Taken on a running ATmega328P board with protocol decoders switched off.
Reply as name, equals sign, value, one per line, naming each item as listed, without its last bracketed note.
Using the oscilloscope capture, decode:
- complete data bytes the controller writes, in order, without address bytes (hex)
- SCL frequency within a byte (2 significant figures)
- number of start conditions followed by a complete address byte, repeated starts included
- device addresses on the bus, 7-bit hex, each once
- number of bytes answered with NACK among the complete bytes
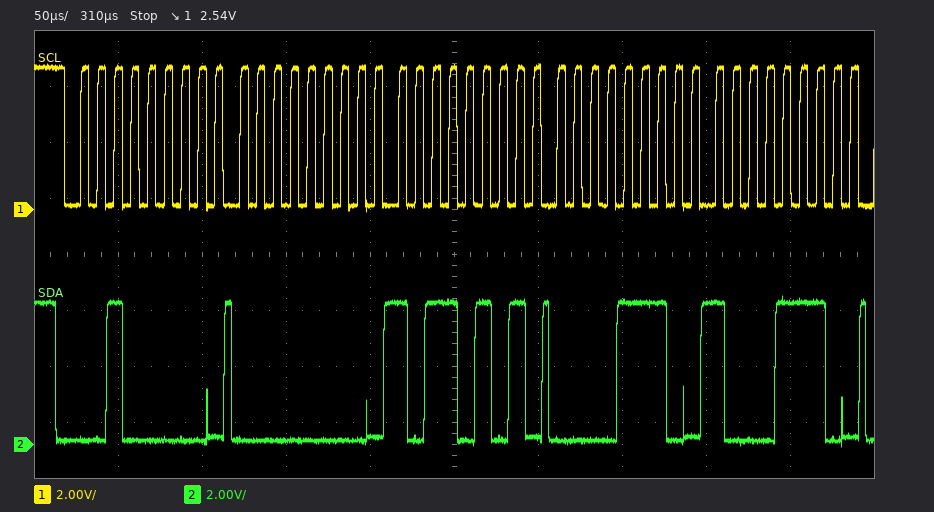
complete data bytes the controller writes, in order, without address bytes = 00 B5 0E 8E
SCL frequency within a byte = 100 kHz
number of start conditions followed by a complete address byte, repeated starts included = 1
device addresses on the bus, 7-bit hex, each once = 0x10
number of bytes answered with NACK among the complete bytes = 0
